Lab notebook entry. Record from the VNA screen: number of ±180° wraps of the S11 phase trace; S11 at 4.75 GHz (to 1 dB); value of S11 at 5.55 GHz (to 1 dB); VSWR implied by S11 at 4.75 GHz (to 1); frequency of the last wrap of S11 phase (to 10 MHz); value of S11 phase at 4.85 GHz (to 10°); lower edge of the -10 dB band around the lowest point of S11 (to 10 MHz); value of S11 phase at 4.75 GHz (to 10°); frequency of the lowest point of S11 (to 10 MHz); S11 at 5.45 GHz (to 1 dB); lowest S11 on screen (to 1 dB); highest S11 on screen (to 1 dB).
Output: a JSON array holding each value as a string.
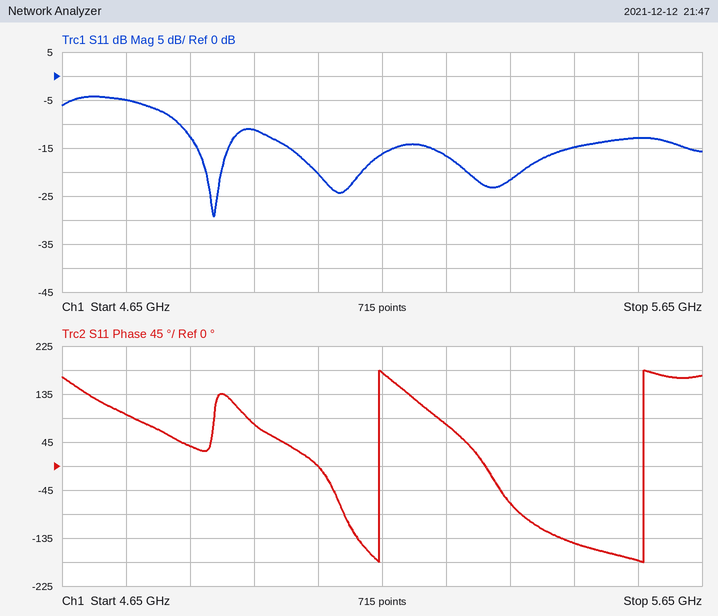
["2", "-5 dB", "-13 dB", "4", "5.56 GHz", "40°", "4.83 GHz", "100°", "4.89 GHz", "-15 dB", "-29 dB", "-4 dB"]
